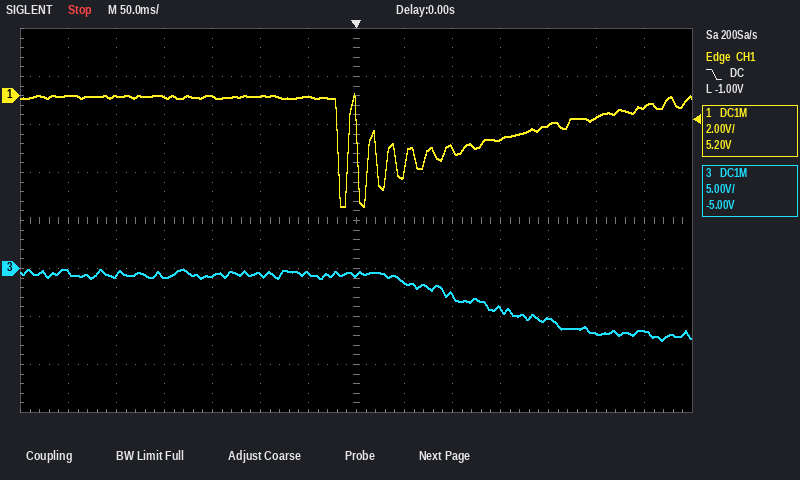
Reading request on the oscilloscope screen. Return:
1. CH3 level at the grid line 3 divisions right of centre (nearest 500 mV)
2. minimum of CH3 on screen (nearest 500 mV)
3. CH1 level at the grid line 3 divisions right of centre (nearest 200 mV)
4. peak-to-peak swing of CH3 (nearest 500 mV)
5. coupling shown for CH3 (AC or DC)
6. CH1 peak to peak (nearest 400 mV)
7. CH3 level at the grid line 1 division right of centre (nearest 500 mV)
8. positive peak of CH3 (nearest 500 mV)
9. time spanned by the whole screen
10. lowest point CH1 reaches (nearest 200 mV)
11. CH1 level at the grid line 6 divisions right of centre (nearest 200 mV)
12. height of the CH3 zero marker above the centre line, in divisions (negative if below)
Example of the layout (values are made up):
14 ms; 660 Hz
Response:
-4.0 V; -7.5 V; -1.8 V; 7.5 V; DC; 4.8 V; -1.5 V; 0.0 V; 700 ms; -4.6 V; -400 mV; -1.0 div
